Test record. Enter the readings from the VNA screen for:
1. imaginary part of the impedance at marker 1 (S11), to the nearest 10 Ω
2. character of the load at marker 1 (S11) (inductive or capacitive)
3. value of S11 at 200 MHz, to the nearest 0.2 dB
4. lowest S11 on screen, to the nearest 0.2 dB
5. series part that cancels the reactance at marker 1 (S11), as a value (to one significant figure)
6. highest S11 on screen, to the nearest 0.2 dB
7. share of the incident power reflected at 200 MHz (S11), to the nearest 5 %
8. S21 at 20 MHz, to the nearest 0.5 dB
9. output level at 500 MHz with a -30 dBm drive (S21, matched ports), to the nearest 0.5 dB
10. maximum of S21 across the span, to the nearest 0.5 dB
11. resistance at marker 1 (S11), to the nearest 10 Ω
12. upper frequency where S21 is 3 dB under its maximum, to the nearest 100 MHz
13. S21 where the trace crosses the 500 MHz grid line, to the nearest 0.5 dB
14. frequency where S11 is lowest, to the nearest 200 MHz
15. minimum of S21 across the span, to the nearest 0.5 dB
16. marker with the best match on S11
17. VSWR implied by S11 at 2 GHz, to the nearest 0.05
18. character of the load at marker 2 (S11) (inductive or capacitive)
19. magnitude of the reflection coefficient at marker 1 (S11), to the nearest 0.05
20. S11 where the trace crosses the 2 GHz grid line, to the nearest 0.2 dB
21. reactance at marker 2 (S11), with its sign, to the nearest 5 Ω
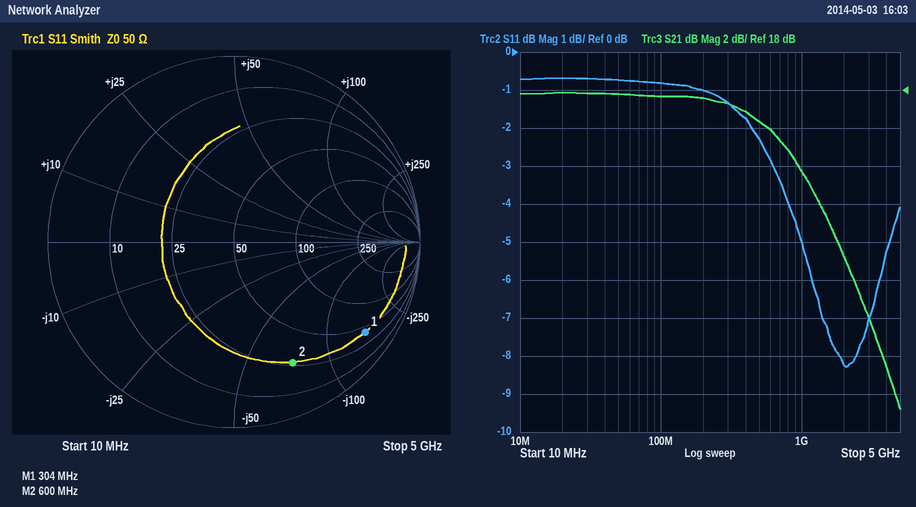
-150 Ω
capacitive
-1.0 dB
-8.2 dB
80 nH
-0.6 dB
80 %
18.0 dB
-13.5 dBm
18.0 dB
40 Ω
800 MHz
16.5 dB
2.0 GHz
1.0 dB
marker 2
2.25
capacitive
0.85
-8.2 dB
-75 Ω
